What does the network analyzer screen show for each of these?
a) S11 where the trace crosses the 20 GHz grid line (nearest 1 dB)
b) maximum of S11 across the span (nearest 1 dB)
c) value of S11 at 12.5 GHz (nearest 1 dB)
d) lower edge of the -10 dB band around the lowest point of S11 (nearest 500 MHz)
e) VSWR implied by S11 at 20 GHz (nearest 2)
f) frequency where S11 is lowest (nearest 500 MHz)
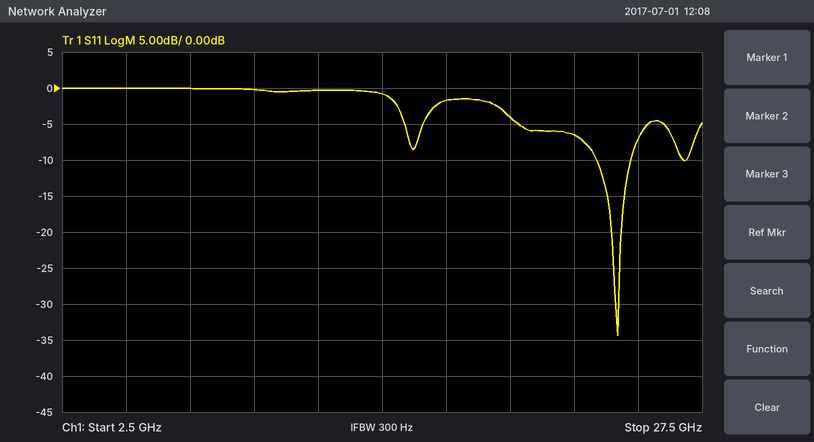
-4 dB
0 dB
0 dB
23.5 GHz
4
24.0 GHz
